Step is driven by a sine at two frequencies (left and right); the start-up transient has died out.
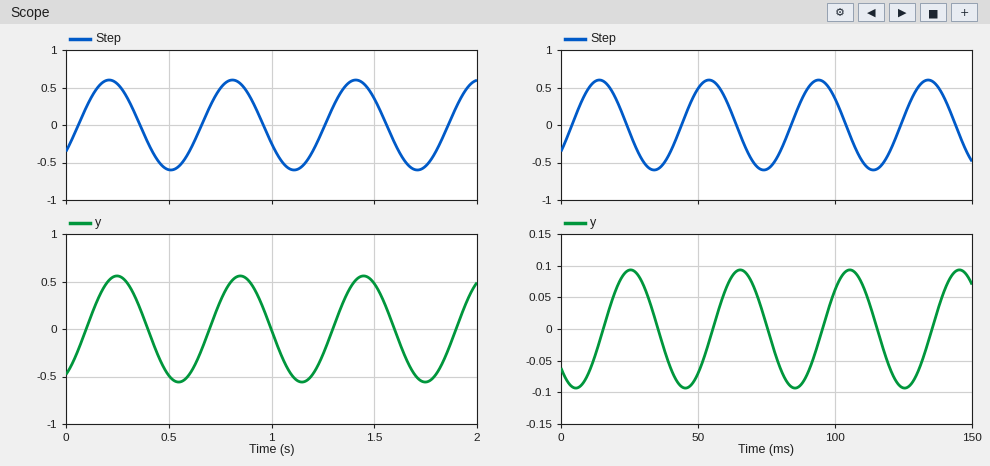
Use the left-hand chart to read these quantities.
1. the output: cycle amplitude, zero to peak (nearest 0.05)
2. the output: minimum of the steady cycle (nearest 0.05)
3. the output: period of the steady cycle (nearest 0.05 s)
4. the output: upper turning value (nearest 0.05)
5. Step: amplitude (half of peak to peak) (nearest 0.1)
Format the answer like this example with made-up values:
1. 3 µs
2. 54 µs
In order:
1. 0.55
2. -0.55
3. 0.60 s
4. 0.55
5. 0.6
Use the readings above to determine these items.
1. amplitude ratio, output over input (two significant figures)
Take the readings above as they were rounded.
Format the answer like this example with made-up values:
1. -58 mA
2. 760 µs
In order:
1. 0.92
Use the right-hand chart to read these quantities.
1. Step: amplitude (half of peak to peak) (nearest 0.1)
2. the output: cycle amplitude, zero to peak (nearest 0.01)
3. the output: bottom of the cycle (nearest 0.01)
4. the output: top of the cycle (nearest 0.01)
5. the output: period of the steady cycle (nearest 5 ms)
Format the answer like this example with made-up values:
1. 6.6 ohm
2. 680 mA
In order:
1. 0.6
2. 0.09
3. -0.09
4. 0.09
5. 40 ms
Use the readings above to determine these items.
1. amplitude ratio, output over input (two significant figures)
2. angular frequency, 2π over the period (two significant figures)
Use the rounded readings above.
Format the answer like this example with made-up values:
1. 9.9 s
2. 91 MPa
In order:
1. 0.15
2. 0.16 rad/ms
